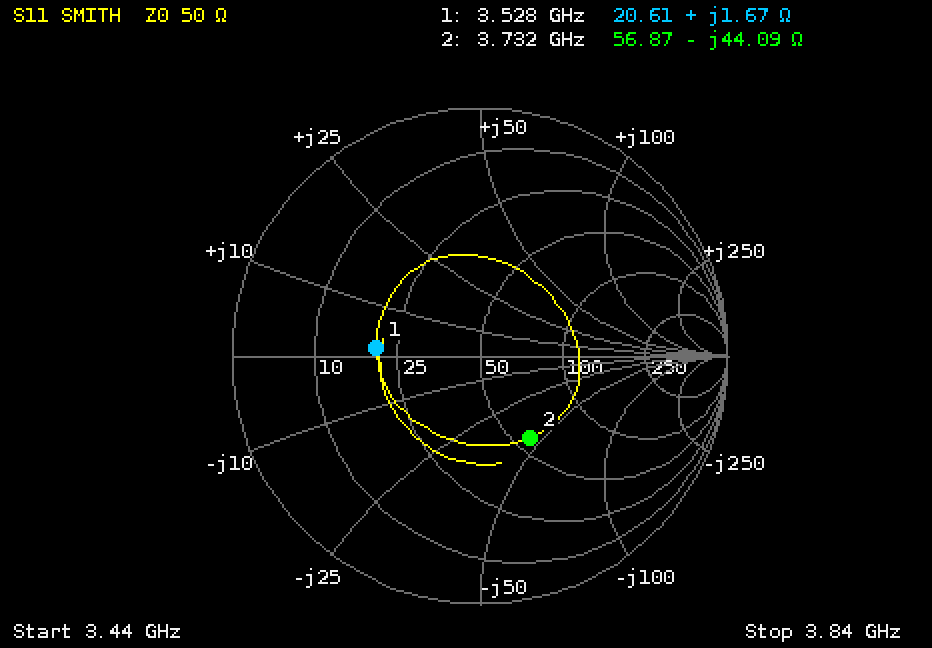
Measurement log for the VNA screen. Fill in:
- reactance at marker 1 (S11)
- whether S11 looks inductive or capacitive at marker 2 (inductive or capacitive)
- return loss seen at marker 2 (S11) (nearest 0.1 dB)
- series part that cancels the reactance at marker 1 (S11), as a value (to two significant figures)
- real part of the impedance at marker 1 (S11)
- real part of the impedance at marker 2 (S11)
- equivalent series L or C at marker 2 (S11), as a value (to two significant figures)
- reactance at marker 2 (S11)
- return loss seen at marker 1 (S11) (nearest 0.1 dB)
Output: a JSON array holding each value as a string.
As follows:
["+1.67 Ω", "capacitive", "8.3 dB", "27 pF", "20.61 Ω", "56.87 Ω", "970 fF", "-44.09 Ω", "7.6 dB"]
